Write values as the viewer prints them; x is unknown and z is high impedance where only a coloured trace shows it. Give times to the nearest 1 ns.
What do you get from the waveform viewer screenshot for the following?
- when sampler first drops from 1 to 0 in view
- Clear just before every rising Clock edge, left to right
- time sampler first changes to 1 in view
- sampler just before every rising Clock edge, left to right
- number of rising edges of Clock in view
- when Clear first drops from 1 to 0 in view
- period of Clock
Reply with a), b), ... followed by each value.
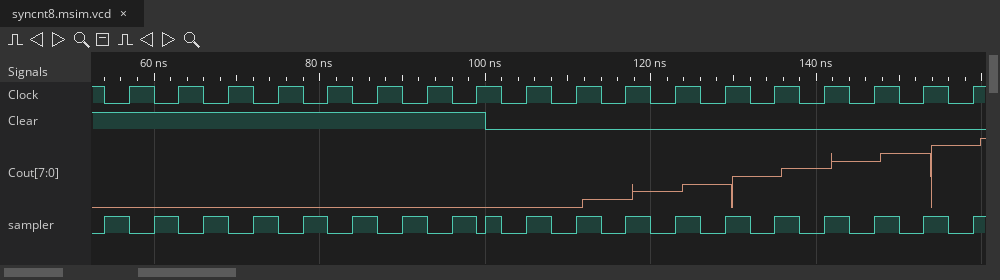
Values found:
a) 57 ns
b) 1 1 1 1 1 1 1 1 0 0 0 0 0 0 0 0 0 0
c) 54 ns
d) 1 1 1 1 1 1 1 1 0 0 0 0 0 0 0 0 0 0
e) 18
f) 100 ns
g) 6 ns
